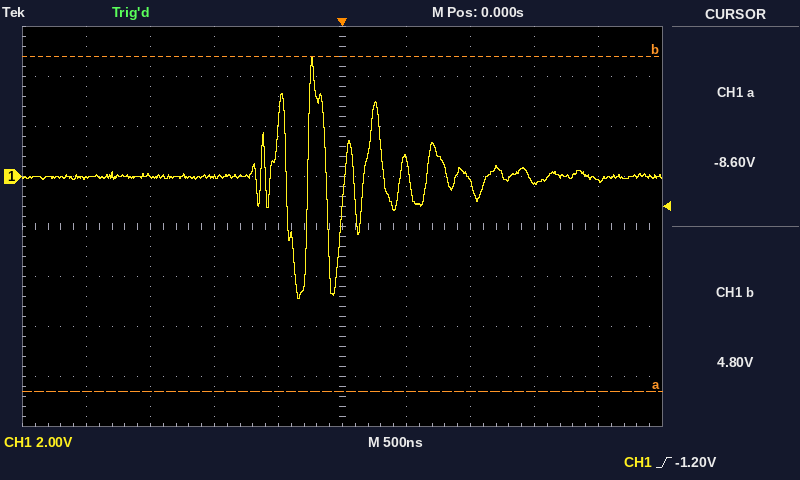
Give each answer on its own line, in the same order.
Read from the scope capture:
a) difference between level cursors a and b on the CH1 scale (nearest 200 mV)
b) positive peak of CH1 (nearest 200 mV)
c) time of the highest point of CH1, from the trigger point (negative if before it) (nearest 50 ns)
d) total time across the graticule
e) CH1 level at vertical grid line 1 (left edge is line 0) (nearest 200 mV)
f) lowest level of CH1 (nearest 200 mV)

13.4 V
4.8 V
-250 ns
5 µs
0.0 V
-4.8 V
